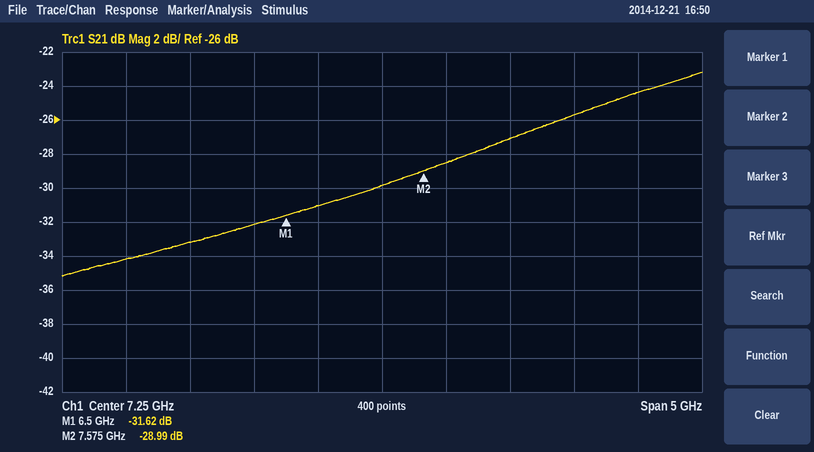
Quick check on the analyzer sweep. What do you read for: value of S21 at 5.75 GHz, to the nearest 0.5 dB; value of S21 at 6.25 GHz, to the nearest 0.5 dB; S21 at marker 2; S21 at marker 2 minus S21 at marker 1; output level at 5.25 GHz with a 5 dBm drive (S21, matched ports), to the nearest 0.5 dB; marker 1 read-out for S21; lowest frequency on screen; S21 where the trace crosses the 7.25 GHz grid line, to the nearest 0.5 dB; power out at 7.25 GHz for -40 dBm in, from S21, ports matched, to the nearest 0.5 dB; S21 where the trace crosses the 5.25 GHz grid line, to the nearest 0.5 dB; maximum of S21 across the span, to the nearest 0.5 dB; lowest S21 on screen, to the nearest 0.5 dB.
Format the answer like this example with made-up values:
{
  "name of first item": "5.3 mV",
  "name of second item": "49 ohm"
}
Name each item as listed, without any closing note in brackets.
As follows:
{
  "value of S21 at 5.75 GHz, to the nearest 0.5 dB": "-33.0 dB",
  "value of S21 at 6.25 GHz, to the nearest 0.5 dB": "-32.0 dB",
  "S21 at marker 2": "-28.99 dB",
  "S21 at marker 2 minus S21 at marker 1": "2.63 dB",
  "output level at 5.25 GHz with a 5 dBm drive (S21, matched ports), to the nearest 0.5 dB": "-29.0 dBm",
  "marker 1 read-out for S21": "-31.62 dB",
  "lowest frequency on screen": "4.75 GHz",
  "S21 where the trace crosses the 7.25 GHz grid line, to the nearest 0.5 dB": "-30.0 dB",
  "power out at 7.25 GHz for -40 dBm in, from S21, ports matched, to the nearest 0.5 dB": "-70.0 dBm",
  "S21 where the trace crosses the 5.25 GHz grid line, to the nearest 0.5 dB": "-34.0 dB",
  "maximum of S21 across the span, to the nearest 0.5 dB": "-23.0 dB",
  "lowest S21 on screen, to the nearest 0.5 dB": "-35.0 dB"
}
